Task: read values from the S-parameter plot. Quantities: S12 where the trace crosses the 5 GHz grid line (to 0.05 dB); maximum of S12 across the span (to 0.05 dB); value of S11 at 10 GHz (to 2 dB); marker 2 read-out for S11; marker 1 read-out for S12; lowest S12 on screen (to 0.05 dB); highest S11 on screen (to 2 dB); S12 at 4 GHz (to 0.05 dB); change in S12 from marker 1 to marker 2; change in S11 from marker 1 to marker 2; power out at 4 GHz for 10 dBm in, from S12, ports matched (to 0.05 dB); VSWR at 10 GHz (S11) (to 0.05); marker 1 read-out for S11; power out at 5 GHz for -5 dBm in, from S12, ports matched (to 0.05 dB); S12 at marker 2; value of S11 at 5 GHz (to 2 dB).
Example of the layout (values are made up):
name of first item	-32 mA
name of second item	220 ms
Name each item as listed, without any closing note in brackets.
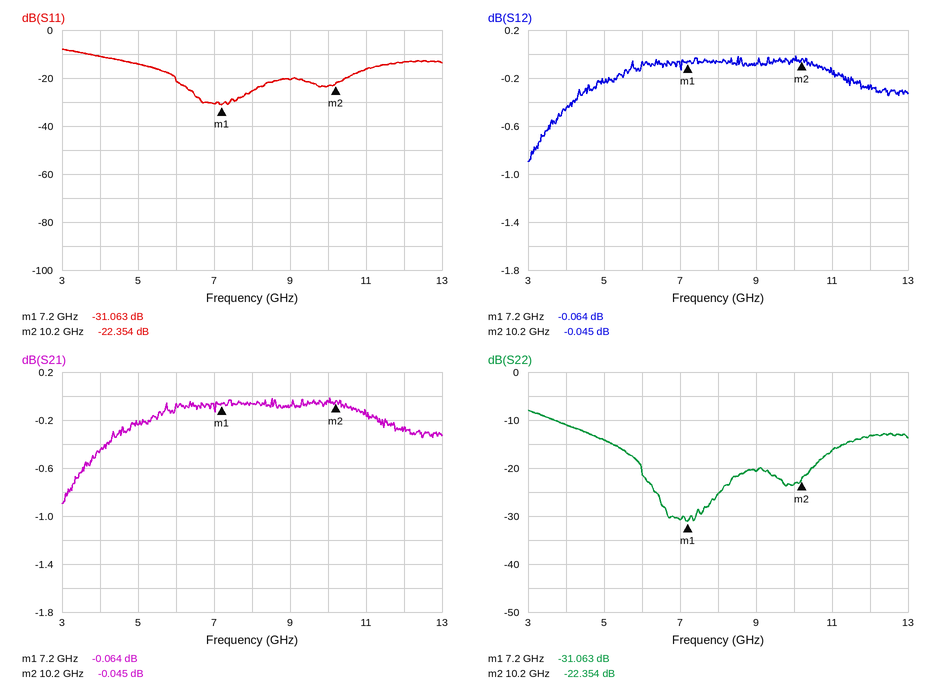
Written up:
S12 where the trace crosses the 5 GHz grid line	-0.25 dB
maximum of S12 across the span	0.00 dB
value of S11 at 10 GHz	-24 dB
marker 2 read-out for S11	-22.354 dB
marker 1 read-out for S12	-0.064 dB
lowest S12 on screen	-0.90 dB
highest S11 on screen	-8 dB
S12 at 4 GHz	-0.45 dB
change in S12 from marker 1 to marker 2	0.019 dB
change in S11 from marker 1 to marker 2	8.709 dB
power out at 4 GHz for 10 dBm in, from S12, ports matched	9.55 dBm
VSWR at 10 GHz (S11)	1.15
marker 1 read-out for S11	-31.063 dB
power out at 5 GHz for -5 dBm in, from S12, ports matched	-5.25 dBm
S12 at marker 2	-0.045 dB
value of S11 at 5 GHz	-14 dB
